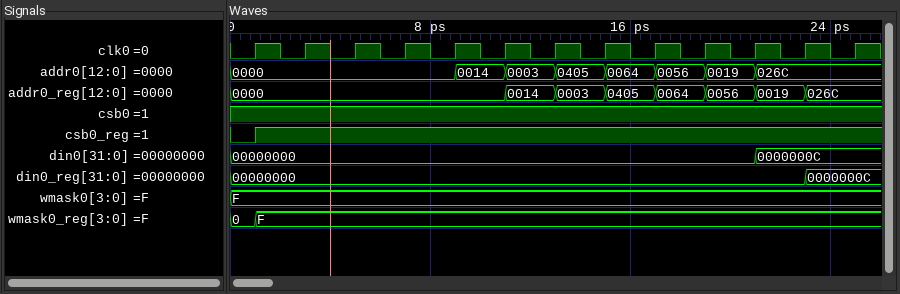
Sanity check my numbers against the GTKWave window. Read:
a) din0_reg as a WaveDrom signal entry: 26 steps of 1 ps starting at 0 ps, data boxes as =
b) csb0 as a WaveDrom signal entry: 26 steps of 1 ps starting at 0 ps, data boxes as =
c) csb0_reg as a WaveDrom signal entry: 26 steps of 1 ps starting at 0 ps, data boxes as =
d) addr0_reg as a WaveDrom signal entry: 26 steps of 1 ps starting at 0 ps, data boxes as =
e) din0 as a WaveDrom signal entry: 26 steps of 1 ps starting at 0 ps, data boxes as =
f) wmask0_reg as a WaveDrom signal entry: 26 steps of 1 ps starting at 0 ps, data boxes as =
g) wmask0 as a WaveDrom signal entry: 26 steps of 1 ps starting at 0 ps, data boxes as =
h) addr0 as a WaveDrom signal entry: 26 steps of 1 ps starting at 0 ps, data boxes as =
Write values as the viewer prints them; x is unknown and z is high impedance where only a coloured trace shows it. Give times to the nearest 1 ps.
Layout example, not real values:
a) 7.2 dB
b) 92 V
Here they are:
a) {name: 'din0_reg', wave: '=......................=..', data: '00000000 0000000C'}
b) {name: 'csb0', wave: '1.........................'}
c) {name: 'csb0_reg', wave: '01........................'}
d) {name: 'addr0_reg', wave: '=..........=.=.=.=.=.=.=..', data: '0000 0014 0003 0405 0064 0056 0019 026C'}
e) {name: 'din0', wave: '=....................=....', data: '00000000 0000000C'}
f) {name: 'wmask0_reg', wave: '==........................', data: '0 F'}
g) {name: 'wmask0', wave: '=.........................', data: 'F'}
h) {name: 'addr0', wave: '=........=.=.=.=.=.=.=....', data: '0000 0014 0003 0405 0064 0056 0019 026C'}
